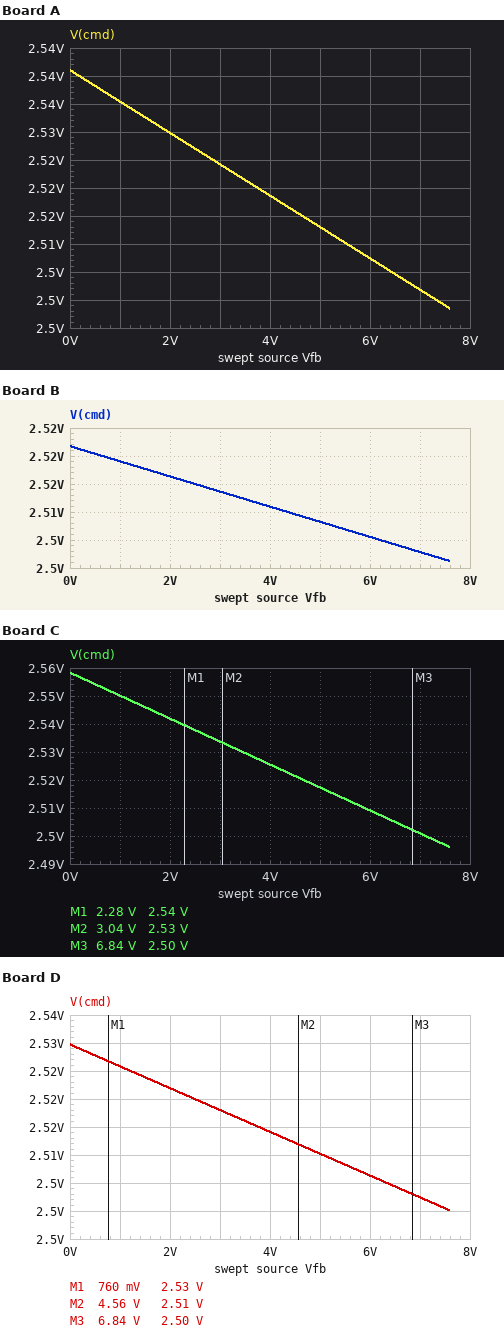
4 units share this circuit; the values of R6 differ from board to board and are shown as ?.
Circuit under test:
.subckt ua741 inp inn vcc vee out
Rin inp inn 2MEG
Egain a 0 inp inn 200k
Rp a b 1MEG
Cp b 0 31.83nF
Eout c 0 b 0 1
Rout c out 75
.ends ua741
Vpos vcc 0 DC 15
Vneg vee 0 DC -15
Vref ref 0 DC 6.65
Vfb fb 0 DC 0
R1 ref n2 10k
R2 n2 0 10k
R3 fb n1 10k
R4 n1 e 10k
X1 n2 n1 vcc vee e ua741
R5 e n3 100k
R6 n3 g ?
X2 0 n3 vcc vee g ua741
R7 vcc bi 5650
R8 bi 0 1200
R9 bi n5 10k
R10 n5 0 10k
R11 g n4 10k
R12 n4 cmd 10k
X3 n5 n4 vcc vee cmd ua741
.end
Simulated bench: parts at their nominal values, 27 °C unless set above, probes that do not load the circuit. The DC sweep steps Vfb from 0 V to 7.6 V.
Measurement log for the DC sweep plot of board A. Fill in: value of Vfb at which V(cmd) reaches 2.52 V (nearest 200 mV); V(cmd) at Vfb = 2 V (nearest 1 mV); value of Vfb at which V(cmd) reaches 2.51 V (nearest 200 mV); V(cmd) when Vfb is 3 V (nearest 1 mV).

3.8 V
2.530 V
5.6 V
2.524 V
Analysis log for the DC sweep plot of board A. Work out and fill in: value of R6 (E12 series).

560 Ω
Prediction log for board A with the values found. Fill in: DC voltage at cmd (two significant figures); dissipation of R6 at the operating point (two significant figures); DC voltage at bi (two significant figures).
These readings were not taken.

2.5 V
2.5 µW
2.5 V
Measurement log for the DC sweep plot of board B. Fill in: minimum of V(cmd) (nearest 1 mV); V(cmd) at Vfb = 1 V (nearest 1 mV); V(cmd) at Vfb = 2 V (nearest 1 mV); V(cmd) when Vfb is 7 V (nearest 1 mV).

2.501 V
2.519 V
2.516 V
2.503 V
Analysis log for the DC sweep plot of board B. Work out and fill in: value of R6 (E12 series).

270 Ω
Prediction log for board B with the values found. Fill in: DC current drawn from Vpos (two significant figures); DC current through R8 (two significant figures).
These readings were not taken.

2.2 mA
2.1 mA
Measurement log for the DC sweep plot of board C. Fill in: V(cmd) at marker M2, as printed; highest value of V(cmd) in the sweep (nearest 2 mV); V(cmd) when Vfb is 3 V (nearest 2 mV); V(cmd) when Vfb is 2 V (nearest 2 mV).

2.53 V
2.558 V
2.534 V
2.542 V
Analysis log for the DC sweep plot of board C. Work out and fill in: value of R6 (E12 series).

820 Ω
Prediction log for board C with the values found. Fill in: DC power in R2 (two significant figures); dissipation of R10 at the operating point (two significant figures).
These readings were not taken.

1.1 mW
160 µW
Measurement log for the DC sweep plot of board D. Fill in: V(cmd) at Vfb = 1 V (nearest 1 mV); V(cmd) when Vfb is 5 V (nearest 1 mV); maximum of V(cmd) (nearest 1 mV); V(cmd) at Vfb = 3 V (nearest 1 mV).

2.526 V
2.510 V
2.530 V
2.518 V
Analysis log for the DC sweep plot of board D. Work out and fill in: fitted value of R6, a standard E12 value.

390 Ω
